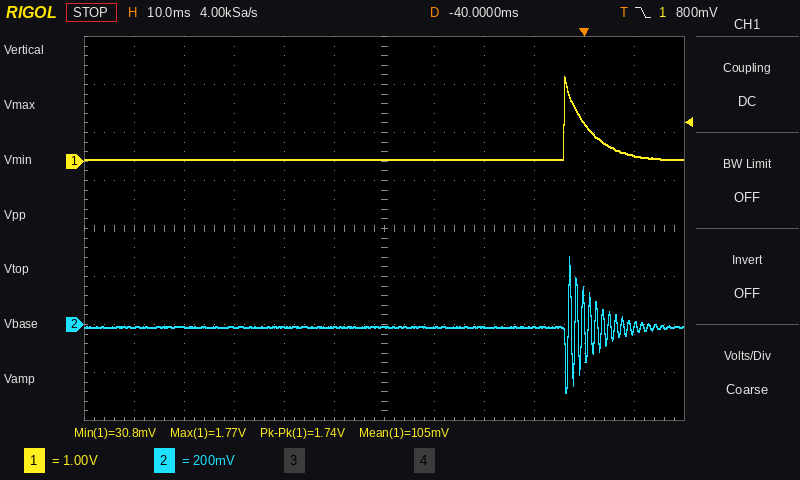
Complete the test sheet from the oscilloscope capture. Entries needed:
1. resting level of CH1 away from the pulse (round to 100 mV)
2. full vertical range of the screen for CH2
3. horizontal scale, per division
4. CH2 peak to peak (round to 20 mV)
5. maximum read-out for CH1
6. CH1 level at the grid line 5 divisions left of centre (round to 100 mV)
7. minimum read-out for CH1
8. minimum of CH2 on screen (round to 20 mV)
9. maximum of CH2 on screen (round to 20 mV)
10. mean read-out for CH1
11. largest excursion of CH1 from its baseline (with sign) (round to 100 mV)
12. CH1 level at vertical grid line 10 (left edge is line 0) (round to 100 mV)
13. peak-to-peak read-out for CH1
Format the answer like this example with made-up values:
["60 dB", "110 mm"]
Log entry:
["0.0 V", "1.6 V", "10 ms", "560 mV", "1.77 V", "0.0 V", "30.8 mV", "-280 mV", "280 mV", "105 mV", "+1.7 V", "800 mV", "1.74 V"]
